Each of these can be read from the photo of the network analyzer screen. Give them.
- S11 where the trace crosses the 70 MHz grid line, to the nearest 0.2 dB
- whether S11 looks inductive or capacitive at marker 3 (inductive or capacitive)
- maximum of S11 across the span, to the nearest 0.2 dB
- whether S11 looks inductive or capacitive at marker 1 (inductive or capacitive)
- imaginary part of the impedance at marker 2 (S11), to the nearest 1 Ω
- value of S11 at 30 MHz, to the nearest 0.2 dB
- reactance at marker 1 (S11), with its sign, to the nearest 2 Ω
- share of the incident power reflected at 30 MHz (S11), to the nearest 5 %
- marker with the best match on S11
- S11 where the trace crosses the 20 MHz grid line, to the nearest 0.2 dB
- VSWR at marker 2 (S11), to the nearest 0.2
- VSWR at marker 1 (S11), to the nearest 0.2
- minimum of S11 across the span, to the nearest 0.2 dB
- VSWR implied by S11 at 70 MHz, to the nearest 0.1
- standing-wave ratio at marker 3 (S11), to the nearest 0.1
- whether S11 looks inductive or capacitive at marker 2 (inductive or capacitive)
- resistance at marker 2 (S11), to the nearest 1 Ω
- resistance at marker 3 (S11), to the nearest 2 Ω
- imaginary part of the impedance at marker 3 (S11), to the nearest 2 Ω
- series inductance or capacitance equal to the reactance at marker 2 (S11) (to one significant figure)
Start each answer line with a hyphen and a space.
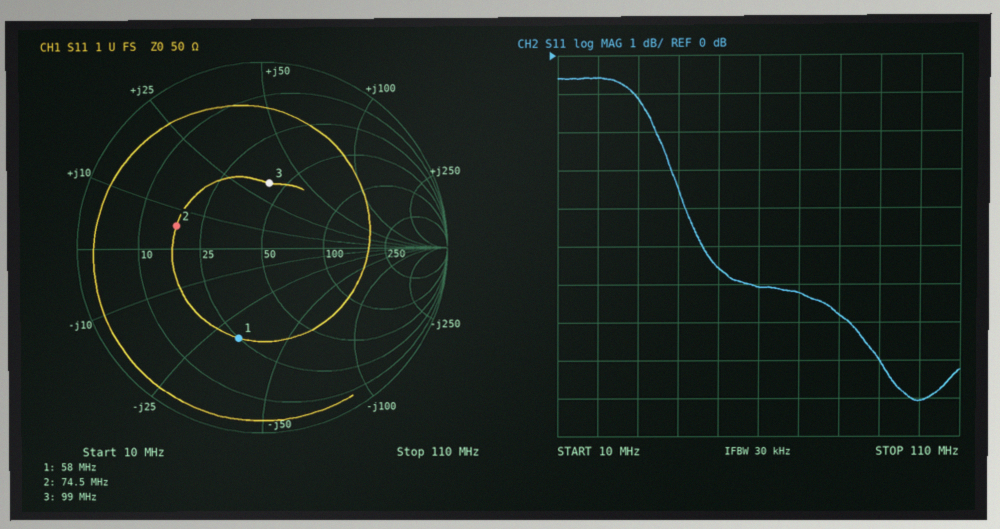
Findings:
- -6.2 dB
- inductive
- -0.6 dB
- capacitive
- +6 Ω
- -1.2 dB
- -32 Ω
- 75 %
- marker 3
- -0.6 dB
- 2.8
- 3.0
- -9.0 dB
- 2.9
- 2.1
- inductive
- 18 Ω
- 42 Ω
- +34 Ω
- 10 nH
